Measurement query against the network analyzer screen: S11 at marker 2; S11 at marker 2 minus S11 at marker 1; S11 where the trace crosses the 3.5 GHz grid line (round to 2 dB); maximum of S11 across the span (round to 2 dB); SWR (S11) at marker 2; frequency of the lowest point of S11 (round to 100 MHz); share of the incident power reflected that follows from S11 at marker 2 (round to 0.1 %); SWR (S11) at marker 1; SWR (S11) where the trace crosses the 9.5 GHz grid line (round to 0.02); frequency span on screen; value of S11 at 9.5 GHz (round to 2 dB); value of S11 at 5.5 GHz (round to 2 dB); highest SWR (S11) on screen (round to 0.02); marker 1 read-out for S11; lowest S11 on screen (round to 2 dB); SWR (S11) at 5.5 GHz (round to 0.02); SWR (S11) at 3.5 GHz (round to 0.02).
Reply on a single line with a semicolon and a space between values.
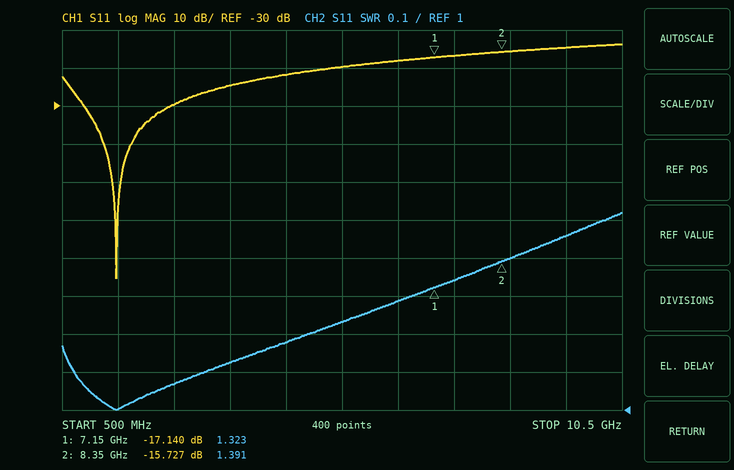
-15.727 dB; 1.413 dB; -24 dB; -14 dB; 1.391; 1.5 GHz; 2.7 %; 1.323; 1.46; 10 GHz; -14 dB; -20 dB; 1.52; -17.140 dB; -76 dB; 1.24; 1.12
